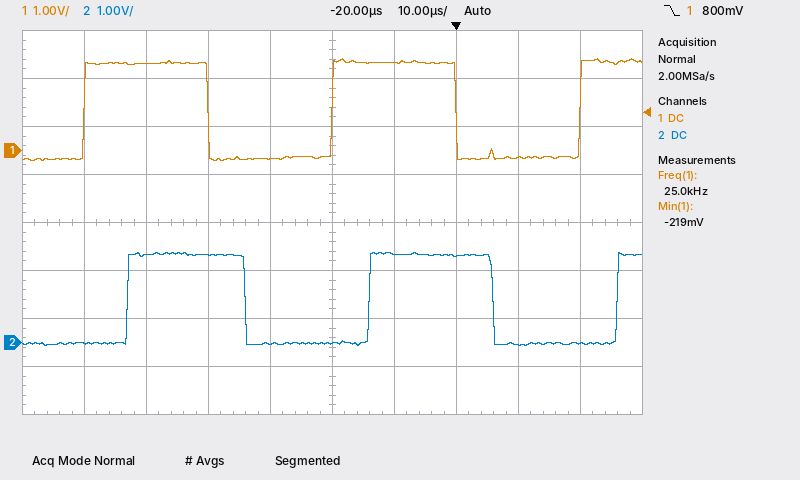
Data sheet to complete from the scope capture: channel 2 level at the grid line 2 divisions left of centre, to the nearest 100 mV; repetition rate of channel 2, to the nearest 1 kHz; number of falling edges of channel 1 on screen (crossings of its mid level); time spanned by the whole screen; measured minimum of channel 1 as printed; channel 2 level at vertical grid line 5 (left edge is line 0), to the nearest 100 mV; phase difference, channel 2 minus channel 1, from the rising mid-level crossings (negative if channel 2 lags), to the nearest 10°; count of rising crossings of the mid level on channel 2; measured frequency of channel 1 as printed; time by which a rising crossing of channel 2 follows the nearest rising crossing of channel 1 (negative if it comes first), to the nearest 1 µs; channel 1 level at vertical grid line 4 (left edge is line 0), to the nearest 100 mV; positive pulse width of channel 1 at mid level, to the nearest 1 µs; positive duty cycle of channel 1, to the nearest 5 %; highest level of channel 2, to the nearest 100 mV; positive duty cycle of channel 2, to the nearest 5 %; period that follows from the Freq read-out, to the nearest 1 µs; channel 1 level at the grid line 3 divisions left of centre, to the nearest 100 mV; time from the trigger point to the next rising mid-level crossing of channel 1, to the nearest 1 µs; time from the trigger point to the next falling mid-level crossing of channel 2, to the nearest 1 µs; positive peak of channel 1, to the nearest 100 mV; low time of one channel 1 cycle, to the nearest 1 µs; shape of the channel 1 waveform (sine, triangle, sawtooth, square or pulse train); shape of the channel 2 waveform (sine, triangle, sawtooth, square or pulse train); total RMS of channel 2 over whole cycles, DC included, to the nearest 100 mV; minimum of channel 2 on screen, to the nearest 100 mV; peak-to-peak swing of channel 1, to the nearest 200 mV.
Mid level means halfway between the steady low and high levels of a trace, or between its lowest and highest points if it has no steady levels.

1.8 V
25 kHz
2
100 µs
-219 mV
0.0 V
-60°
3
25.0 kHz
+6 µs
-200 mV
20 µs
50 %
1.9 V
50 %
40 µs
1.8 V
20 µs
6 µs
1.9 V
20 µs
square
square
1.3 V
-100 mV
2.2 V
